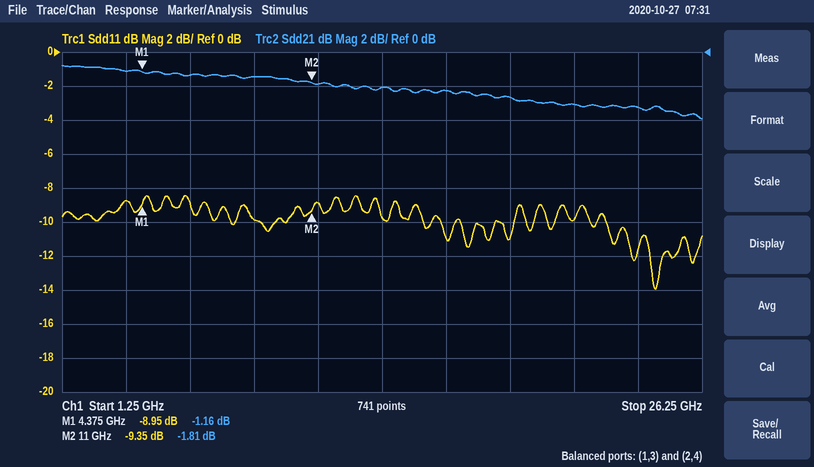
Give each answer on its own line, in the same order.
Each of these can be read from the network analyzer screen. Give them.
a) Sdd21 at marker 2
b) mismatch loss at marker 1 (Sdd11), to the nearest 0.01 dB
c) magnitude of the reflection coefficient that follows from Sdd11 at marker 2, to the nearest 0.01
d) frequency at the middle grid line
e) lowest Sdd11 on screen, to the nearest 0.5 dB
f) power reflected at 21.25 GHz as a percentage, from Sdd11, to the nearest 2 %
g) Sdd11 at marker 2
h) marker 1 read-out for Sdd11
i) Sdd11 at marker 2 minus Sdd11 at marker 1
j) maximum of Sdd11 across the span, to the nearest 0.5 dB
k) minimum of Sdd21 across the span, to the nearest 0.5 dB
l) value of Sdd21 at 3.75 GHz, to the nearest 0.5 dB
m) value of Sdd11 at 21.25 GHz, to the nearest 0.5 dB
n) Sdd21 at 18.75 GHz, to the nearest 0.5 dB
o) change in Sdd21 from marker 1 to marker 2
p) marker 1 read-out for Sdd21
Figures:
-1.81 dB
0.59 dB
0.34
13.75 GHz
-14.0 dB
10 %
-9.35 dB
-8.95 dB
-0.40 dB
-8.5 dB
-4.0 dB
-1.0 dB
-10.0 dB
-2.5 dB
-0.65 dB
-1.16 dB
